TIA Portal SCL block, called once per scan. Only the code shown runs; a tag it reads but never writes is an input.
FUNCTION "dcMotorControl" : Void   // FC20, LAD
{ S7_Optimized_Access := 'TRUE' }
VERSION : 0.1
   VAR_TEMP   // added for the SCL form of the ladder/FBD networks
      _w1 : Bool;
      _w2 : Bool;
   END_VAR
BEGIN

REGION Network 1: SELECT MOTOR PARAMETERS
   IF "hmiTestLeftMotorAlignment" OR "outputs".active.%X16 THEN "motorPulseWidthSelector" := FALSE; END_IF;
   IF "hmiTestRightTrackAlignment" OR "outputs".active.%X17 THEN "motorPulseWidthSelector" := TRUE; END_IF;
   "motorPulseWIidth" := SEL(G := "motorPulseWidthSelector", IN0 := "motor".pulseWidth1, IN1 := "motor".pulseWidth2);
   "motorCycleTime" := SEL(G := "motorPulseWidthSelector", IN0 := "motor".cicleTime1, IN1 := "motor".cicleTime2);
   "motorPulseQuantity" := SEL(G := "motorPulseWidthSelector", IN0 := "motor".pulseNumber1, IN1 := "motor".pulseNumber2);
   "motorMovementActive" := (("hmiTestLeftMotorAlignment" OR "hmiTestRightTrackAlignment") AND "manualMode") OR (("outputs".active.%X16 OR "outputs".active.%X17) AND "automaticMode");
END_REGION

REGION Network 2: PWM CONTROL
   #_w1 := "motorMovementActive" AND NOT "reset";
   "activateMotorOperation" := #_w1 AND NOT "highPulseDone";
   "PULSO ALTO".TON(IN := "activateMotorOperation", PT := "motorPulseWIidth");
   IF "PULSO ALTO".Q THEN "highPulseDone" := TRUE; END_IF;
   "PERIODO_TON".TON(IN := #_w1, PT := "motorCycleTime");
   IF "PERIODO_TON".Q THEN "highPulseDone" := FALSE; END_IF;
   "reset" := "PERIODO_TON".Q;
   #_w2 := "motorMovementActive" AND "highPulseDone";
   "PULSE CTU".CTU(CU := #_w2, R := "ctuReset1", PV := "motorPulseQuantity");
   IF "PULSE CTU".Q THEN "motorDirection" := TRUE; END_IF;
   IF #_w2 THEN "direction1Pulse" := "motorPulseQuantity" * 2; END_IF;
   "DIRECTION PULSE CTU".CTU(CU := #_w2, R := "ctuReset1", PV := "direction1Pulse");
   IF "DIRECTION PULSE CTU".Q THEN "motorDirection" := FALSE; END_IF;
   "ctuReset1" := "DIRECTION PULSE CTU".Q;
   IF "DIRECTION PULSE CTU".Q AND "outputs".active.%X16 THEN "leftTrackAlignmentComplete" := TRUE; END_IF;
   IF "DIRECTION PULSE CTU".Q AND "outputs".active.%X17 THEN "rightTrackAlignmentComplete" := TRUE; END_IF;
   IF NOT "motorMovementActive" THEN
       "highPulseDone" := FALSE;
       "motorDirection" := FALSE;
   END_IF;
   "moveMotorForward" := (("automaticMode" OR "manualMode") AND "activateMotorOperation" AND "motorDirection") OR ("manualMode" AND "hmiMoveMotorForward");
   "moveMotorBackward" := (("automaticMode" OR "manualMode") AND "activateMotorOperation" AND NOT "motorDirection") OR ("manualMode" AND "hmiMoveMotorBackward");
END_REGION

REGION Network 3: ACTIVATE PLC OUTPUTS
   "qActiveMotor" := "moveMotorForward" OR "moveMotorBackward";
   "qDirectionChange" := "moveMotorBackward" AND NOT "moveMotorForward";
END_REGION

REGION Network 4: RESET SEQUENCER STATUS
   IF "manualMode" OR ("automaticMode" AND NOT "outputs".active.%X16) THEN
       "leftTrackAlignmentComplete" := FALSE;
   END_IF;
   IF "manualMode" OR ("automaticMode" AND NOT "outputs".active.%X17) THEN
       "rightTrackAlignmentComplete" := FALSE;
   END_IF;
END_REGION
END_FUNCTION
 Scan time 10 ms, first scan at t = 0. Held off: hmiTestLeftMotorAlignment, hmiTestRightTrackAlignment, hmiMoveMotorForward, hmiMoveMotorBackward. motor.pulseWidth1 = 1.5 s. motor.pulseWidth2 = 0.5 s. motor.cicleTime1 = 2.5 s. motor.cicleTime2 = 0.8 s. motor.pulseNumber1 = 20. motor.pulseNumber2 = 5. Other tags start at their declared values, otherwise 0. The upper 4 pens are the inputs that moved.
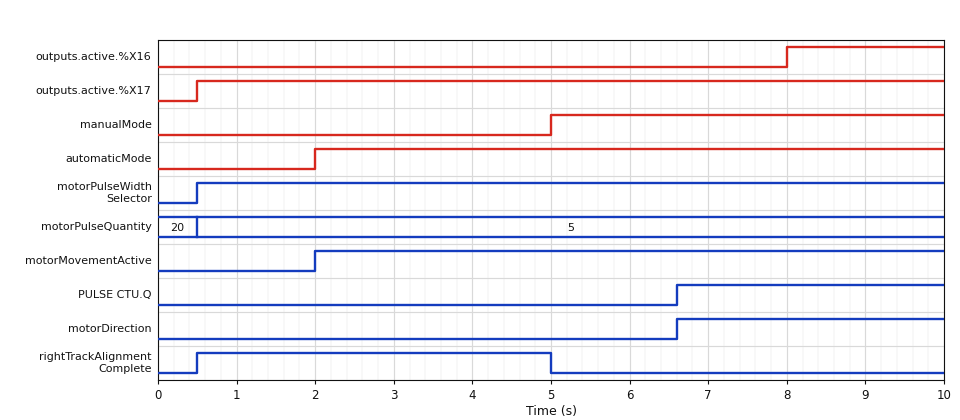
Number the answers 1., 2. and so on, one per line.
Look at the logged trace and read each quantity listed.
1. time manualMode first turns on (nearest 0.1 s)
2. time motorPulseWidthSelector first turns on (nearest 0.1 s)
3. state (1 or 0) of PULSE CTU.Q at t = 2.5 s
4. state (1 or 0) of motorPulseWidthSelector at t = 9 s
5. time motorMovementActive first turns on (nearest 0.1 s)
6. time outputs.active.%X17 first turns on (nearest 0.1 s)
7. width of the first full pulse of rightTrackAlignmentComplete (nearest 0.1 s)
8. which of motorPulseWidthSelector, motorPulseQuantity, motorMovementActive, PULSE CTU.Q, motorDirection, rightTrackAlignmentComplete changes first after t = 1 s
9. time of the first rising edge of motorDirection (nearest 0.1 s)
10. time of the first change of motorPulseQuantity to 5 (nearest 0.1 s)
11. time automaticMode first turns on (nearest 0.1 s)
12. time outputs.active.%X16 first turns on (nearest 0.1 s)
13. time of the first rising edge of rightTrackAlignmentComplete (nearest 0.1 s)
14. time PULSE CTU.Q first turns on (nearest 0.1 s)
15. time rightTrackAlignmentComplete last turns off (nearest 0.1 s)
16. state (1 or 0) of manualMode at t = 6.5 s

1. 5.0 s
2. 0.5 s
3. 0
4. 1
5. 2.0 s
6. 0.5 s
7. 4.5 s
8. motorMovementActive
9. 6.6 s
10. 0.5 s
11. 2.0 s
12. 8.0 s
13. 0.5 s
14. 6.6 s
15. 5.0 s
16. 1
